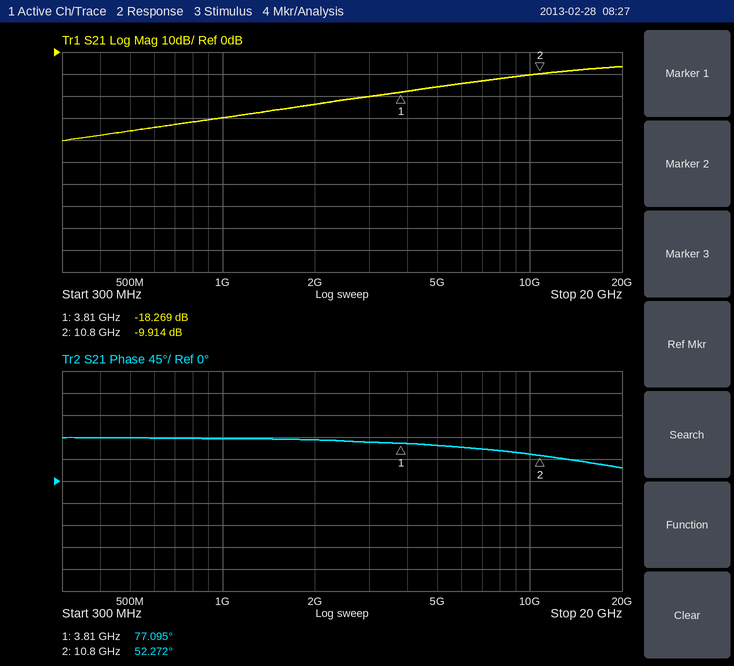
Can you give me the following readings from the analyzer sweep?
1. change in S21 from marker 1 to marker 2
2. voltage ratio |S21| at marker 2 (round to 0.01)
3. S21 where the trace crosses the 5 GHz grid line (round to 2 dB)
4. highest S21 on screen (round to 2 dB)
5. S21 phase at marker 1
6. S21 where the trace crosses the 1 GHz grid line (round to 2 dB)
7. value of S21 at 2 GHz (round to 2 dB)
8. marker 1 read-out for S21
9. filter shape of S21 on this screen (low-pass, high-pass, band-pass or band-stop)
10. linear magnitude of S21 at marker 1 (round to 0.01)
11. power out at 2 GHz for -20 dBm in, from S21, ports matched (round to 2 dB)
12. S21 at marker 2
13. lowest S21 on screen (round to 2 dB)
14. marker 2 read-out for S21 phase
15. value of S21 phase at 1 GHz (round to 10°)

8.355 dB
0.32
-16 dB
-6 dB
77.095°
-30 dB
-24 dB
-18.269 dB
high-pass
0.12
-44 dBm
-9.914 dB
-40 dB
52.272°
90°
